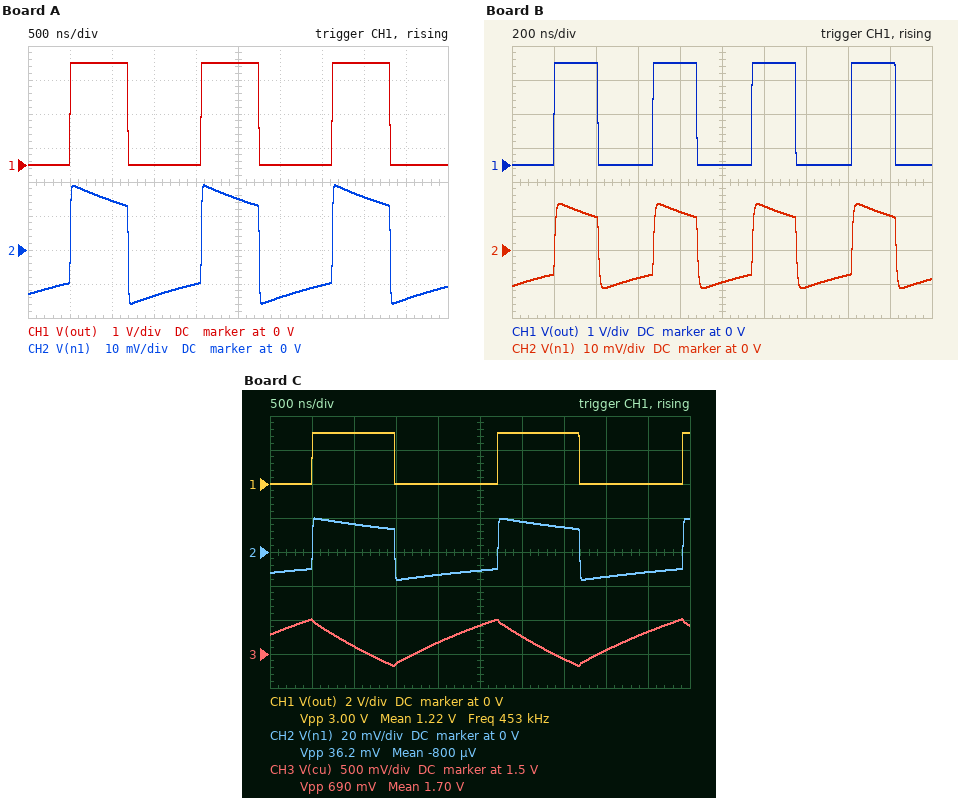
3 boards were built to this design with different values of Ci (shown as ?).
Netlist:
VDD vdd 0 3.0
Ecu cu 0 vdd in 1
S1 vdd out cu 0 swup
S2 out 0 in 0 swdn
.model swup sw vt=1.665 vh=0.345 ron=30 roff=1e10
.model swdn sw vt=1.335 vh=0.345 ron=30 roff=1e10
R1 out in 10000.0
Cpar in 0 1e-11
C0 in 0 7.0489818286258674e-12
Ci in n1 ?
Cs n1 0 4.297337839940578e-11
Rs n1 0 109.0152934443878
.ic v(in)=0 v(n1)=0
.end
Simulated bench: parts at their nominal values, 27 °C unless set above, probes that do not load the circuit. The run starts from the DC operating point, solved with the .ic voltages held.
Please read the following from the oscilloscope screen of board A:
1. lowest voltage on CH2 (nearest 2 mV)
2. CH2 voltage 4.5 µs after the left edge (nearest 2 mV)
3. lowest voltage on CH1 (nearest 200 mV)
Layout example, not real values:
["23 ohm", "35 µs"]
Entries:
["-16 mV", "-14 mV", "0 V"]
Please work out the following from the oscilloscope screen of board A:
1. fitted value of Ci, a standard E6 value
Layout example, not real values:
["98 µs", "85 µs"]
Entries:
["150 pF"]
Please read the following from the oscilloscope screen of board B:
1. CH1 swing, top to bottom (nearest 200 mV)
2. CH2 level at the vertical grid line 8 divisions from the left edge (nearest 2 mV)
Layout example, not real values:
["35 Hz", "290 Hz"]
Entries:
["3.0 V", "-8 mV"]
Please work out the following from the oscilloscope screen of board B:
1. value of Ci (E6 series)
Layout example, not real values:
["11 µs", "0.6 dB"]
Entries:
["33 pF"]
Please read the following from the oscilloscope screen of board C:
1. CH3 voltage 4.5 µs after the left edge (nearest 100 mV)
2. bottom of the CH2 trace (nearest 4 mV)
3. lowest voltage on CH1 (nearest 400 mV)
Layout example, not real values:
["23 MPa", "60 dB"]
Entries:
["1.8 V", "-16 mV", "0 V"]
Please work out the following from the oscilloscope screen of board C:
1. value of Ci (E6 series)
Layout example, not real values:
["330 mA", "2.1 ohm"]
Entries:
["220 pF"]
